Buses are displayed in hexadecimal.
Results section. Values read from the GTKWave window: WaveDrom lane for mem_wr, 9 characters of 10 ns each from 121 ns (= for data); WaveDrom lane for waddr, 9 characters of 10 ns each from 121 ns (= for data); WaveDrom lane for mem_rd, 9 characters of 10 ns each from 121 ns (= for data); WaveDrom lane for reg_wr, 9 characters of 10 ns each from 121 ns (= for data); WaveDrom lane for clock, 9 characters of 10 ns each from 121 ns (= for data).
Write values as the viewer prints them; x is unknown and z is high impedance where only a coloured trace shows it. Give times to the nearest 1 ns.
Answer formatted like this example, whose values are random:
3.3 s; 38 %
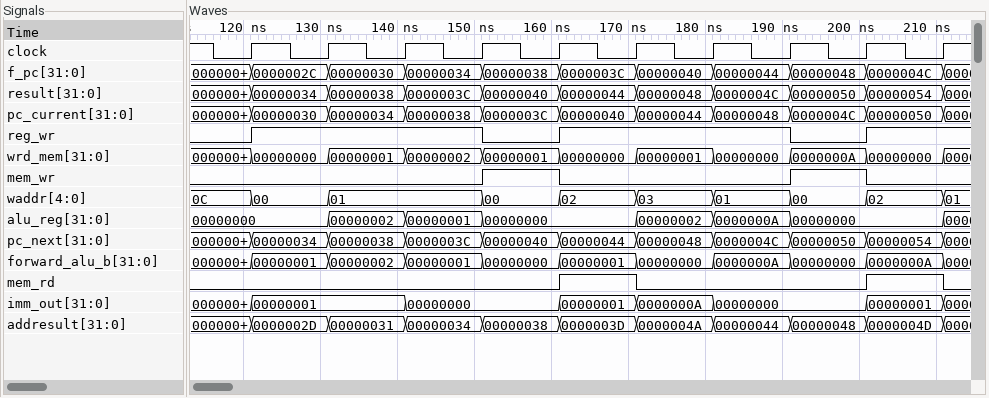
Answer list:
{name: 'mem_wr', wave: '0..10..10'}; {name: 'waddr', wave: '==.======', data: '00 01 00 02 03 01 00 02'}; {name: 'mem_rd', wave: '0...10..1'}; {name: 'reg_wr', wave: '1..01..01'}; {name: 'clock', wave: 'p........'}
